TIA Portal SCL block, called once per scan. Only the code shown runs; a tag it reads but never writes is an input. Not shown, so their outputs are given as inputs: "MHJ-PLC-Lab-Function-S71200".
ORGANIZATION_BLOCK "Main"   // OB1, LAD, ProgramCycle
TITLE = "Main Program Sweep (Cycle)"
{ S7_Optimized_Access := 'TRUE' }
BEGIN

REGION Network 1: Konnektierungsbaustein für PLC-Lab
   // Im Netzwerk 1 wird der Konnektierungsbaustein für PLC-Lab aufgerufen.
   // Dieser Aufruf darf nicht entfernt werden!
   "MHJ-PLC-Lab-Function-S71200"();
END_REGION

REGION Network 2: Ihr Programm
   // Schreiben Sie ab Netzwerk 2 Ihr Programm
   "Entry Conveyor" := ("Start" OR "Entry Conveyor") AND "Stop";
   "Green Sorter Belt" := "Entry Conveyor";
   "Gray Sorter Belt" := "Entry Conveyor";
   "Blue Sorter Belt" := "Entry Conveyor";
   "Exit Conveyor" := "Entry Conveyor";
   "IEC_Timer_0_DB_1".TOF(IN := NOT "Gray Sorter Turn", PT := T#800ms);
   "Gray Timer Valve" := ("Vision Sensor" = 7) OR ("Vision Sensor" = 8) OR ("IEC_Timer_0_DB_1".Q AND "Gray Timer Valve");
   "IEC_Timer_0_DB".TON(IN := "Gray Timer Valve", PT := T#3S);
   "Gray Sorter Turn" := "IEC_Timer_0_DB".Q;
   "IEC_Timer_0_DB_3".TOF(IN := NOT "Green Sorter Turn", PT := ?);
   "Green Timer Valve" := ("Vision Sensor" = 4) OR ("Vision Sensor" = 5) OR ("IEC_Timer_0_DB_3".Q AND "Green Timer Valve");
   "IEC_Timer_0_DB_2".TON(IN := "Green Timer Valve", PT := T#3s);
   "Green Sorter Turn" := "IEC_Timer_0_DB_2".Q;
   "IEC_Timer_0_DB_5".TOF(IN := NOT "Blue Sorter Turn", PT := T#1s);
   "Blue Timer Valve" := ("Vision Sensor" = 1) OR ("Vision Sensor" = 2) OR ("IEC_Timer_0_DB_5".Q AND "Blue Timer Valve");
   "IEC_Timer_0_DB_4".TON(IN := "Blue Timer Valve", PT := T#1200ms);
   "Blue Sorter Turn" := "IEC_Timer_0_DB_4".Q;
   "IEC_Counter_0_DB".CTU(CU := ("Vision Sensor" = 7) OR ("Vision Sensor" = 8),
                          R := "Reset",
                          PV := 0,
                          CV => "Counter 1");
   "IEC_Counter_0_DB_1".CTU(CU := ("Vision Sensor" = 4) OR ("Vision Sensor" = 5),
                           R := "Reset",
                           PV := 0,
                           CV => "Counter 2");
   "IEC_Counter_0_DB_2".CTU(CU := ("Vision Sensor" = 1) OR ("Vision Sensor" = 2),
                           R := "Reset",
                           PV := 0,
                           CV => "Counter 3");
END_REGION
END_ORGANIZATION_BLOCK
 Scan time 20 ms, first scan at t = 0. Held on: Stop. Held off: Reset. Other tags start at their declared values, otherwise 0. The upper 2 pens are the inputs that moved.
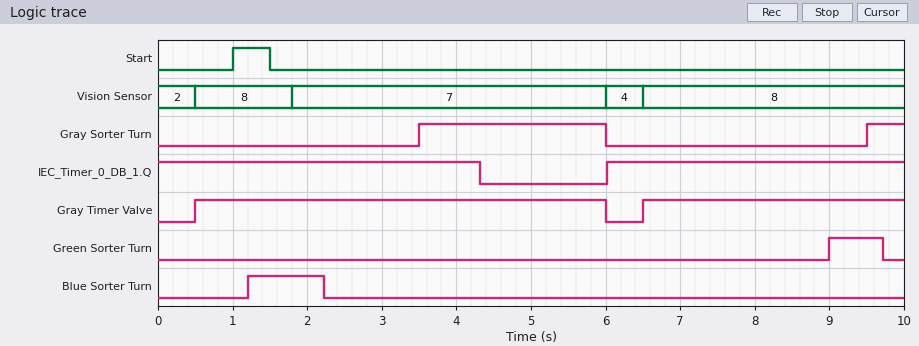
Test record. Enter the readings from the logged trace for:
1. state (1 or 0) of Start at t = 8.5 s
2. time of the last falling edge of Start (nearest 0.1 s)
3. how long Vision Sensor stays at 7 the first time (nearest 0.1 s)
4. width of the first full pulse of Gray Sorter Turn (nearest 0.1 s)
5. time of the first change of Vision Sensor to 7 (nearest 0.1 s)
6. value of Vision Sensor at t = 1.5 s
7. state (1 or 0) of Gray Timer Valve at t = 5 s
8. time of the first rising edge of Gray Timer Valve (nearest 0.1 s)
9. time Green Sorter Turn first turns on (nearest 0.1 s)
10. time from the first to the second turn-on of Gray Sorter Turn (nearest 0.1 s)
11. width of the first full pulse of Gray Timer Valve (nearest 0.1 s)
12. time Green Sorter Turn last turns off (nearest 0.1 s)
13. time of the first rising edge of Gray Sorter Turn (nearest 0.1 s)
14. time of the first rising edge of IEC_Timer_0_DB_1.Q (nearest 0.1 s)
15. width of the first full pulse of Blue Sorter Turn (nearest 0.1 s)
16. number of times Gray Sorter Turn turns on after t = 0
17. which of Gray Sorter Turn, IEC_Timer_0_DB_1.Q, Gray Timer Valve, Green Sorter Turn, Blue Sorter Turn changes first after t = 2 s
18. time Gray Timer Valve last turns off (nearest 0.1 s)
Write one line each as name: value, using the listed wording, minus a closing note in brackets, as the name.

state (1 or 0) of Start at t = 8.5 s: 0
time of the last falling edge of Start: 1.5 s
how long Vision Sensor stays at 7 the first time: 4.2 s
width of the first full pulse of Gray Sorter Turn: 2.5 s
time of the first change of Vision Sensor to 7: 1.8 s
value of Vision Sensor at t = 1.5 s: 8
state (1 or 0) of Gray Timer Valve at t = 5 s: 1
time of the first rising edge of Gray Timer Valve: 0.5 s
time Green Sorter Turn first turns on: 9.0 s
time from the first to the second turn-on of Gray Sorter Turn: 6.0 s
width of the first full pulse of Gray Timer Valve: 5.5 s
time Green Sorter Turn last turns off: 9.7 s
time of the first rising edge of Gray Sorter Turn: 3.5 s
time of the first rising edge of IEC_Timer_0_DB_1.Q: 6.0 s
width of the first full pulse of Blue Sorter Turn: 1.0 s
number of times Gray Sorter Turn turns on after t = 0: 2
which of Gray Sorter Turn, IEC_Timer_0_DB_1.Q, Gray Timer Valve, Green Sorter Turn, Blue Sorter Turn changes first after t = 2 s: Blue Sorter Turn
time Gray Timer Valve last turns off: 6.0 s
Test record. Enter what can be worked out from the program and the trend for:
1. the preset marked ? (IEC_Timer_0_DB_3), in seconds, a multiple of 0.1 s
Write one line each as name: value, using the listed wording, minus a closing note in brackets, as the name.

the preset marked ? (IEC_Timer_0_DB_3), in seconds, a multiple of 0.1 s: 0.7 s
